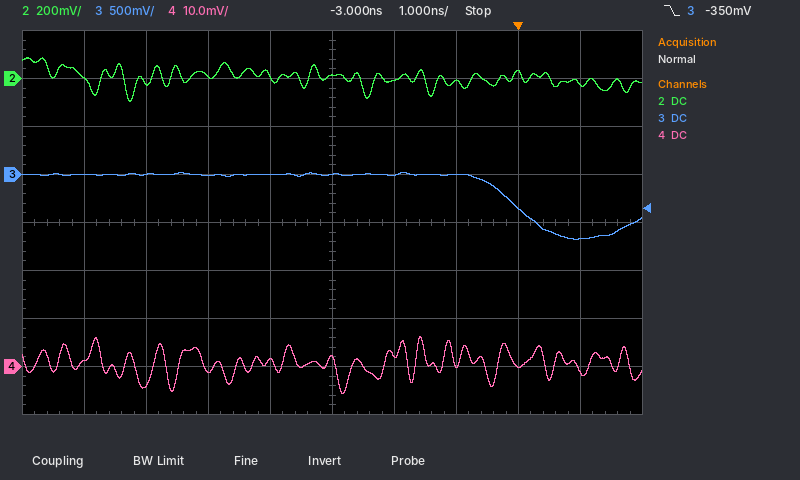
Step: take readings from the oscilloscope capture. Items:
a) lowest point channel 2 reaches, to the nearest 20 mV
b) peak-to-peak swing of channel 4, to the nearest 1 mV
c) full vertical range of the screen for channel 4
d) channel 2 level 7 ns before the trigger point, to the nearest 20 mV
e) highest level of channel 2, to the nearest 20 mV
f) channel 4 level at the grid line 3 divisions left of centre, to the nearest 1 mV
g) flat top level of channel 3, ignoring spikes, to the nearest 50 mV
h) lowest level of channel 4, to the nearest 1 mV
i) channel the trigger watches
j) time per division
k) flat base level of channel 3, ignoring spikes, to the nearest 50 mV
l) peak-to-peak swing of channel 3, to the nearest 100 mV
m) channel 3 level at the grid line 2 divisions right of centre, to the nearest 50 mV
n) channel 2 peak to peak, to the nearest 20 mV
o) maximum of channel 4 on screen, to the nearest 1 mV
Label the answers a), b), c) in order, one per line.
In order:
a) -100 mV
b) 12 mV
c) 80 mV
d) 0 mV
e) 80 mV
f) -4 mV
g) 0 mV
h) -6 mV
i) channel 3
j) 1 ns
k) -650 mV
l) 700 mV
m) 0 mV
n) 180 mV
o) 6 mV
